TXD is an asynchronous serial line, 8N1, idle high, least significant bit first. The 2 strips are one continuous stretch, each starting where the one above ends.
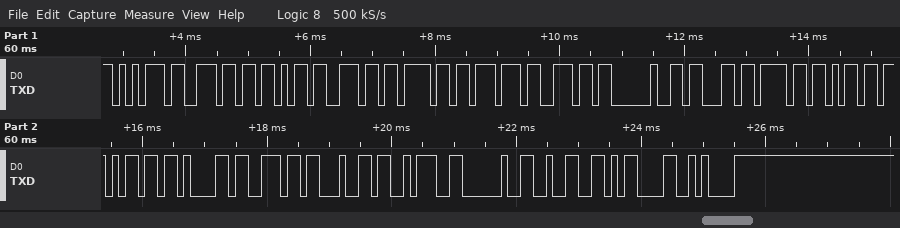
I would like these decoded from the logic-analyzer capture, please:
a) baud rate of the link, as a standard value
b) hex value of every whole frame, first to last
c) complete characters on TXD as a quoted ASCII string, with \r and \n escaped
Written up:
9600 baud
0x75 0x6E 0x6B 0x6E 0x6F 0x77 0x6E 0x20 0x63 0x6F 0x6D 0x6D 0x61 0x6E 0x64 0x3A 0x20 0x32 0x0D 0x0A
"unknown command: 2\r\n"
